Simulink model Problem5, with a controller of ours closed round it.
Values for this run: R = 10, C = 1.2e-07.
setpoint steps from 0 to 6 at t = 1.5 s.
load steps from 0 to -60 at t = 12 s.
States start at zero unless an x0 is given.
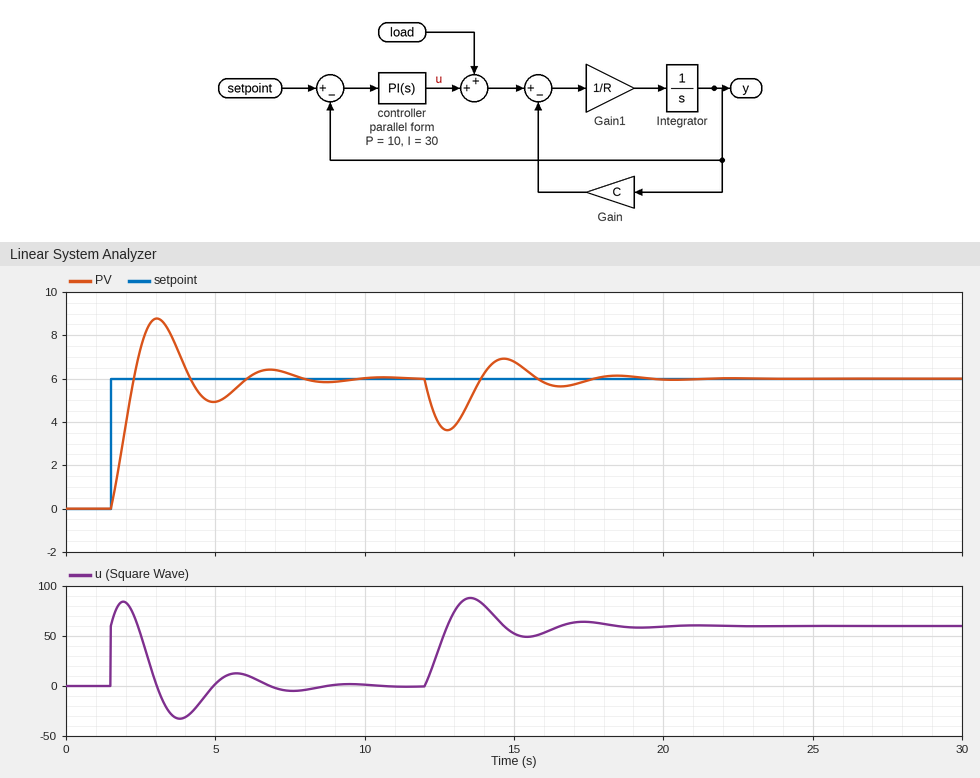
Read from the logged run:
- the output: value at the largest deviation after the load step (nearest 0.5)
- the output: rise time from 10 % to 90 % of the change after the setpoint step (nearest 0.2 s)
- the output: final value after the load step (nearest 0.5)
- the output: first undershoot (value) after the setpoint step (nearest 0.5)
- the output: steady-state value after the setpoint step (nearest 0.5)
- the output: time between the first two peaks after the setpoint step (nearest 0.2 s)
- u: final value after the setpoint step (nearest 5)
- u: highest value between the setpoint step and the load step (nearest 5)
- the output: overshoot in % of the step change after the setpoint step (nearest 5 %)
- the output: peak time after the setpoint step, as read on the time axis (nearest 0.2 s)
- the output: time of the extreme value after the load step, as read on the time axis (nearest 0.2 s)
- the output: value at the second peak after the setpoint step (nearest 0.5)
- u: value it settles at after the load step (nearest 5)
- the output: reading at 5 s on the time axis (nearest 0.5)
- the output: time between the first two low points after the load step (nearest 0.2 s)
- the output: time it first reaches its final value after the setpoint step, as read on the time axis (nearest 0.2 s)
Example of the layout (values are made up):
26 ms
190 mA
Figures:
3.5
0.6 s
6.0
5.0
6.0
3.8 s
0
85
45 %
3.0 s
12.8 s
6.5
60
5.0
3.8 s
2.2 s
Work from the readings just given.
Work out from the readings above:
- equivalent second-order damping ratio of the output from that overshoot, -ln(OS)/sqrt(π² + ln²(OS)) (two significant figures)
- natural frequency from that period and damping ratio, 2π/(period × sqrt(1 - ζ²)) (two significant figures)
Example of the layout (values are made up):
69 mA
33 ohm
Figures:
0.25
1.7 rad/s
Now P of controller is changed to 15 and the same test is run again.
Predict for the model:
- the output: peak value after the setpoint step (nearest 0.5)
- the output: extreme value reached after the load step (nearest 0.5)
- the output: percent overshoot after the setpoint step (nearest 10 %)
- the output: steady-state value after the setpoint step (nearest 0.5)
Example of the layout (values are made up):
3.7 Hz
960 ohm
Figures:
8.0
4.0
30 %
6.0
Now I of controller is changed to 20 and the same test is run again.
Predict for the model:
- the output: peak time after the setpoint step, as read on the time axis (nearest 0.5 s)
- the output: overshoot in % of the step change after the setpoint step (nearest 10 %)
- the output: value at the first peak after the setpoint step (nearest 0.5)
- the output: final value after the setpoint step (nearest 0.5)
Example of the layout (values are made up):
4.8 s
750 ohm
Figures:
3.5 s
40 %
8.5
6.0
